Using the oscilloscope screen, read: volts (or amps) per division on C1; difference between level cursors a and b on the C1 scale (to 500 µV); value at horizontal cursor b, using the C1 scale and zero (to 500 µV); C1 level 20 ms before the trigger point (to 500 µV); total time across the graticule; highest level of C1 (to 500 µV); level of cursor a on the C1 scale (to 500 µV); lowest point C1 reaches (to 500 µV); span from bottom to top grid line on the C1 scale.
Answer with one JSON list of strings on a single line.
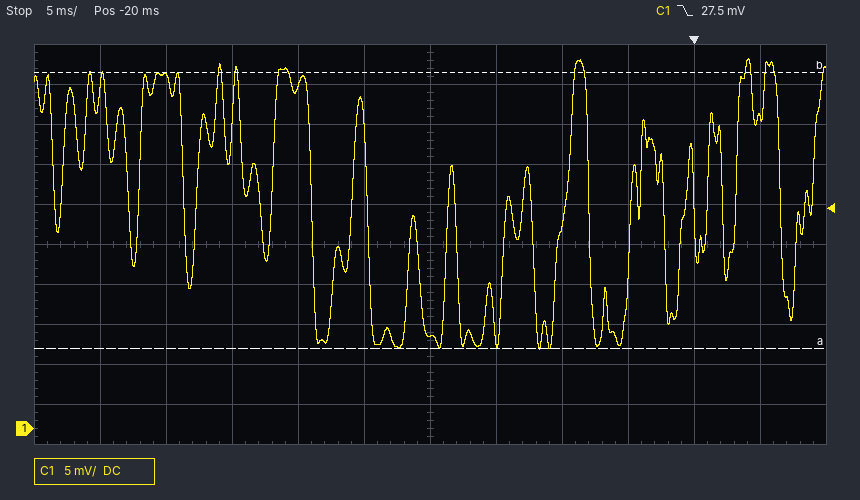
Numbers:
["5 mV", "34.5 mV", "44.5 mV", "11.5 mV", "60 ms", "46.0 mV", "10.0 mV", "10.0 mV", "50 mV"]
